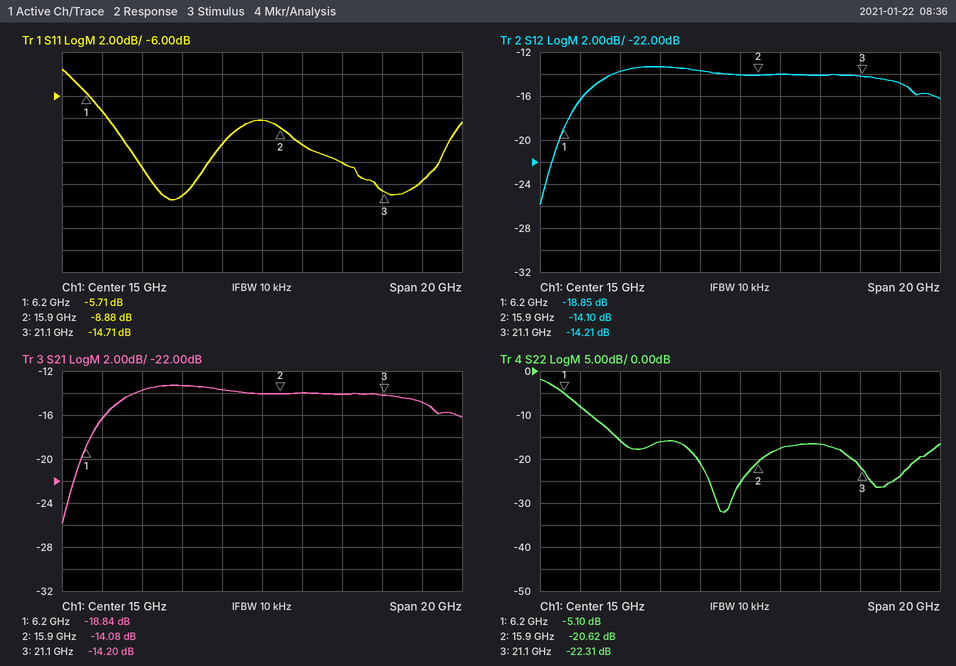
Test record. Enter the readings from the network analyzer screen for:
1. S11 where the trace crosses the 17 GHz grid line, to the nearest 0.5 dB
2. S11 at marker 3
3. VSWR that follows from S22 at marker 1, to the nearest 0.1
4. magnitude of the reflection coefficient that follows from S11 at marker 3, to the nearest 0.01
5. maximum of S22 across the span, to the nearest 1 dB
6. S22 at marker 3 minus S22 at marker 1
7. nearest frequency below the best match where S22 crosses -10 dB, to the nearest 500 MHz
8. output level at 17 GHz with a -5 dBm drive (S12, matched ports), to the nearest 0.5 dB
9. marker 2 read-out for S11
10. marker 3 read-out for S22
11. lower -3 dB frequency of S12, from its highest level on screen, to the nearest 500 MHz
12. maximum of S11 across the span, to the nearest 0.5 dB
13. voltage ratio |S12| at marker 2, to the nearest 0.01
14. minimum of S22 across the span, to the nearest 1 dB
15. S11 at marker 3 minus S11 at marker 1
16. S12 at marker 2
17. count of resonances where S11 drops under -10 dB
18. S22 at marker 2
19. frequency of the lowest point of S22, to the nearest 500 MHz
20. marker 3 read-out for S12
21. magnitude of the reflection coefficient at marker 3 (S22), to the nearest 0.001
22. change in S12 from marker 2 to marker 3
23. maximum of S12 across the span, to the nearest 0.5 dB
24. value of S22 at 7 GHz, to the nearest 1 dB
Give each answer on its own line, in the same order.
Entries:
-10.5 dB
-14.71 dB
3.5
0.18
-2 dB
-17.21 dB
7.5 GHz
-19.0 dBm
-8.88 dB
-22.31 dB
7.0 GHz
-3.5 dB
0.20
-32 dB
-9.00 dB
-14.10 dB
2
-20.62 dB
14.0 GHz
-14.21 dB
0.077
-0.11 dB
-13.5 dB
-8 dB
